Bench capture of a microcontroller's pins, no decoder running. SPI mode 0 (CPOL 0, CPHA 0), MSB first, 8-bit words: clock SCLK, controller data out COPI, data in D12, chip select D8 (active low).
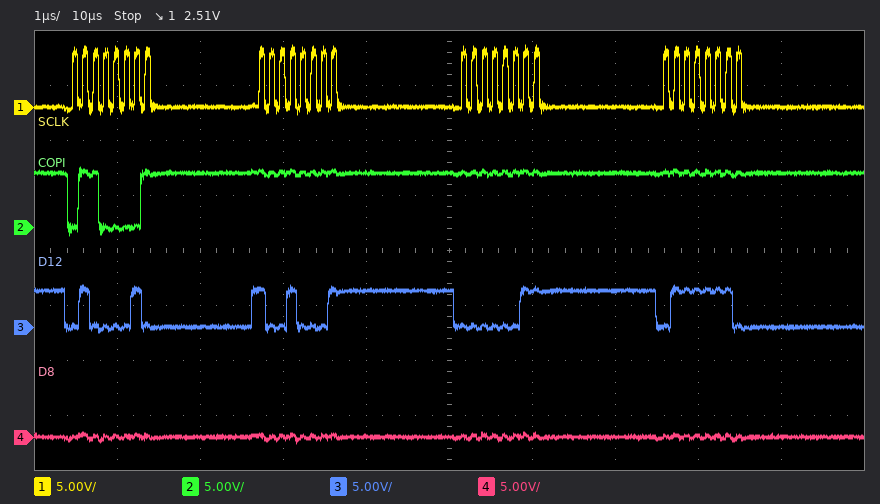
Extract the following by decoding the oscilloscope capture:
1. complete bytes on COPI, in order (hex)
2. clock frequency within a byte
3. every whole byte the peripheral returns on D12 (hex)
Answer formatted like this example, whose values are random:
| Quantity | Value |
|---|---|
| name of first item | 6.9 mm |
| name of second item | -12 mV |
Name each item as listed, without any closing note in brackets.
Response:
| Quantity | Value |
|---|---|
| complete bytes on COPI, in order | 61 FF FF FF |
| clock frequency within a byte | 8 MHz |
| every whole byte the peripheral returns on D12 | 42 91 03 7E |
